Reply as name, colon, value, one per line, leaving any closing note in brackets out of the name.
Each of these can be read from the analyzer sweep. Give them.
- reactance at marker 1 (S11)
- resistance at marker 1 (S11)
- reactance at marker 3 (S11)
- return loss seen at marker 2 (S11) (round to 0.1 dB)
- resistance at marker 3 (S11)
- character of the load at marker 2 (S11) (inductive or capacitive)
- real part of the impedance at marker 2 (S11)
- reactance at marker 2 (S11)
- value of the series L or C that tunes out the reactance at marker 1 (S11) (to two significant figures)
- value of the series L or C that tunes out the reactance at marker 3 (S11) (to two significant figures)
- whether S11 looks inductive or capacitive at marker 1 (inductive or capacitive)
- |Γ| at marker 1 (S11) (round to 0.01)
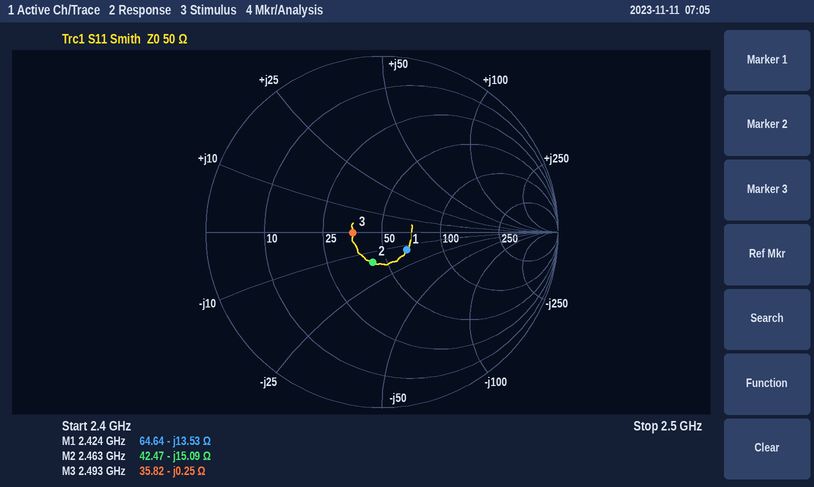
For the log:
reactance at marker 1: -13.53 Ω
resistance at marker 1: 64.64 Ω
reactance at marker 3: -0.25 Ω
return loss seen at marker 2 (S11): 14.9 dB
resistance at marker 3: 35.82 Ω
character of the load at marker 2 (S11): capacitive
real part of the impedance at marker 2: 42.47 Ω
reactance at marker 2: -15.09 Ω
value of the series L or C that tunes out the reactance at marker 1 (S11): 890 pH
value of the series L or C that tunes out the reactance at marker 3 (S11): 16 pH
whether S11 looks inductive or capacitive at marker 1: capacitive
|Γ| at marker 1 (S11): 0.17
